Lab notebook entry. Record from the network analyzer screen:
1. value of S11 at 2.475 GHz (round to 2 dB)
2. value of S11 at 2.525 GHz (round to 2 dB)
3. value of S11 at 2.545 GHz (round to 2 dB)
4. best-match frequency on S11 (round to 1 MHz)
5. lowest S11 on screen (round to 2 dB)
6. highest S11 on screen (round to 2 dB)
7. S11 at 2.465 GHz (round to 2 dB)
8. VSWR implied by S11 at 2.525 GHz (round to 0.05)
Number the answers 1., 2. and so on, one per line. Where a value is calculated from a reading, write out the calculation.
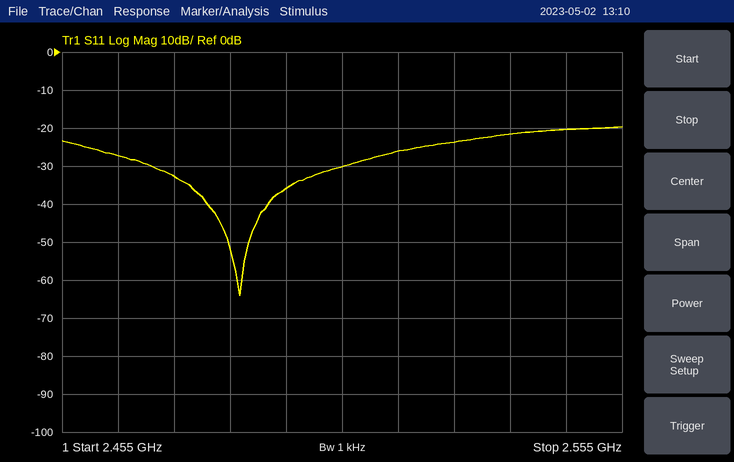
1. -32 dB
2. -24 dB
3. -20 dB
4. 2.487 GHz
5. -64 dB
6. -20 dB
7. -28 dB
8. |Γ| = 10^(-24/20) = 0.0631; VSWR = (1 + 0.0631)/(1 − 0.0631) ≈ 1.13, so 1.15 to the nearest 0.05
